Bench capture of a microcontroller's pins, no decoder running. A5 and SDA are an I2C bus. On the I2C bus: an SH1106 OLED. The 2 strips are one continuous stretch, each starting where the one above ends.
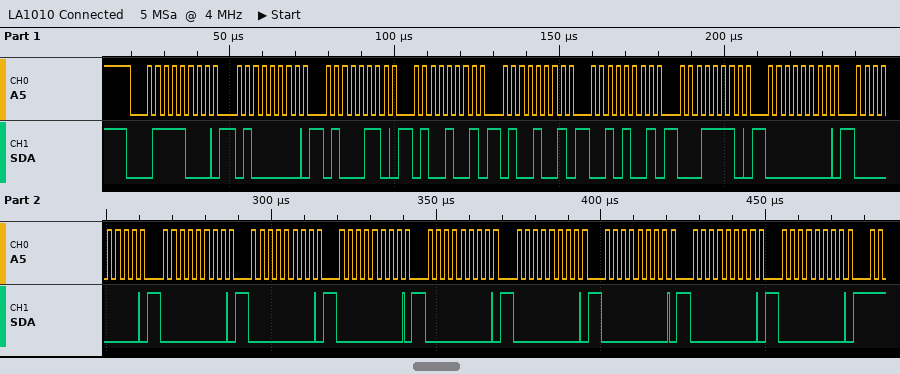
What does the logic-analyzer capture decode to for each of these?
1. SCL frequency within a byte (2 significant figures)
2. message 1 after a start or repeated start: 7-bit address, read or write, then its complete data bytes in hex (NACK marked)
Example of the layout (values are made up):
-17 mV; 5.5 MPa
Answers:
400 kHz; 0x3C write: 40 46 49 49 29 1E 00 00 00 00 00 00 00 00 00 00
